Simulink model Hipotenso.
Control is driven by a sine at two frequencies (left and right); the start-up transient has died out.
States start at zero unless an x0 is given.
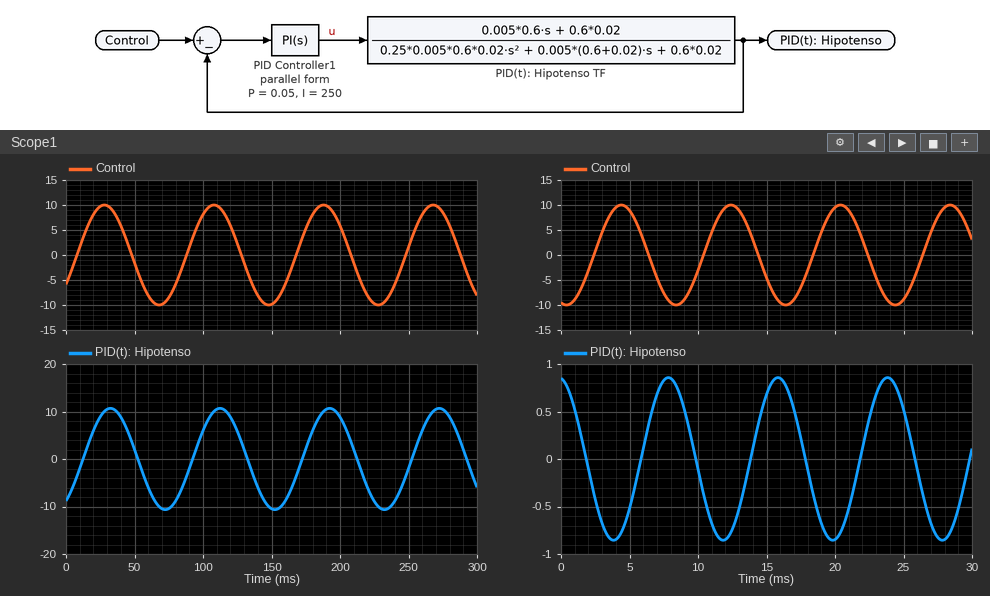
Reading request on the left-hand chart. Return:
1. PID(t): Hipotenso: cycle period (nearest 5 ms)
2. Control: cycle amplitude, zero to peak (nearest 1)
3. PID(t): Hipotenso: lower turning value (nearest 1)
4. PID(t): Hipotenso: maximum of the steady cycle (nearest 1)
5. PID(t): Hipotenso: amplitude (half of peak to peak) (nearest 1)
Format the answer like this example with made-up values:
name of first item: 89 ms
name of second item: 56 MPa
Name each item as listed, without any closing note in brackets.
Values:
PID(t): Hipotenso: cycle period: 80 ms
Control: cycle amplitude, zero to peak: 10
PID(t): Hipotenso: lower turning value: -11
PID(t): Hipotenso: maximum of the steady cycle: 11
PID(t): Hipotenso: amplitude (half of peak to peak): 11
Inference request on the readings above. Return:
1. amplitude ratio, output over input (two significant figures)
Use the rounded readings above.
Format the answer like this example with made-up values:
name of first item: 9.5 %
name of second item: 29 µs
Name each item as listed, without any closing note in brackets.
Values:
amplitude ratio, output over input: 1.1
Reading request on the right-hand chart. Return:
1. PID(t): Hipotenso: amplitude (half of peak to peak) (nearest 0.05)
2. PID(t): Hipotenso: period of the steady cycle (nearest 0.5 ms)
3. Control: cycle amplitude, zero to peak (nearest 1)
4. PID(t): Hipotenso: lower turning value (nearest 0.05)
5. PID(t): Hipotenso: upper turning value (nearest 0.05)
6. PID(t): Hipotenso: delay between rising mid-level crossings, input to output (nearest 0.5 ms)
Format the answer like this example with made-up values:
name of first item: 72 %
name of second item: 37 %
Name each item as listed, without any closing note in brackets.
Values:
PID(t): Hipotenso: amplitude (half of peak to peak): 0.85
PID(t): Hipotenso: period of the steady cycle: 8.0 ms
Control: cycle amplitude, zero to peak: 10
PID(t): Hipotenso: lower turning value: -0.85
PID(t): Hipotenso: upper turning value: 0.85
PID(t): Hipotenso: delay between rising mid-level crossings, input to output: 3.5 ms
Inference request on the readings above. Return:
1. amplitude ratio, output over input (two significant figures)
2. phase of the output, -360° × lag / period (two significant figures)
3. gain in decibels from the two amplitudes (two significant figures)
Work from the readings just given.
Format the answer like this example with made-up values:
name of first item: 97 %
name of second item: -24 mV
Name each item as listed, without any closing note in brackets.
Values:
amplitude ratio, output over input: 0.085
phase of the output, -360° × lag / period: -160°
gain in decibels from the two amplitudes: -21 dB
